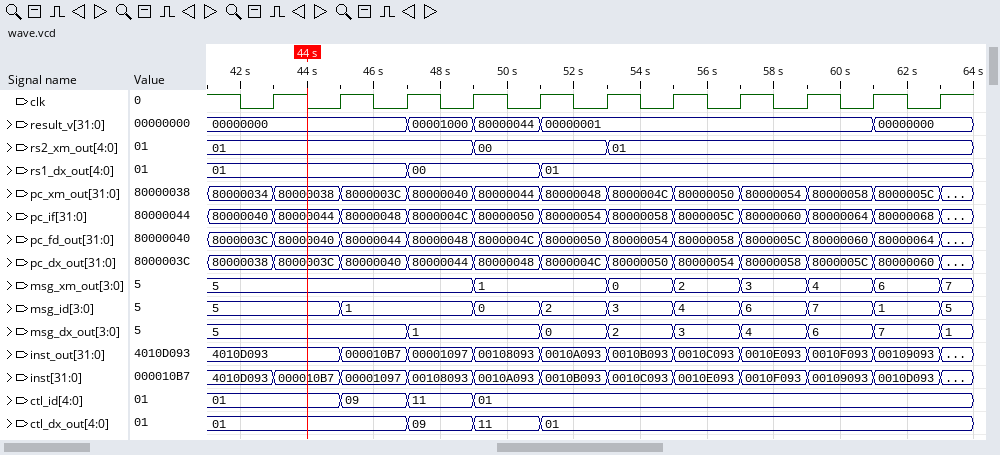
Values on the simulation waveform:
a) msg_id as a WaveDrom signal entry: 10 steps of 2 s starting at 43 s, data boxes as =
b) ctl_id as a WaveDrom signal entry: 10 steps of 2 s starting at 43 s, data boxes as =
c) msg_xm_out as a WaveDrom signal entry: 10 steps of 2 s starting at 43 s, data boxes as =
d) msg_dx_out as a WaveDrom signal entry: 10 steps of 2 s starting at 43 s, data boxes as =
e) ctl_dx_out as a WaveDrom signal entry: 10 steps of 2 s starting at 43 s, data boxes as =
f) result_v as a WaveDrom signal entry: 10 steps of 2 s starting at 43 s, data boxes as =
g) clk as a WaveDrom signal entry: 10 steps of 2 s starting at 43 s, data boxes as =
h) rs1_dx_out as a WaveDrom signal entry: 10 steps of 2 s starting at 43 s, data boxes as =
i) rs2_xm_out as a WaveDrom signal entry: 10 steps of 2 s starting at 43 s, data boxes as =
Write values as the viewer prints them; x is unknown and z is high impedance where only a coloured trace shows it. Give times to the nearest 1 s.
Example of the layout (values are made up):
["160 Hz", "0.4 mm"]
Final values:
["{name: 'msg_id', wave: '==.=======', data: '5 1 0 2 3 4 6 7 1'}", "{name: 'ctl_id', wave: '====......', data: '01 09 11 01'}", "{name: 'msg_xm_out', wave: '=..=.=====', data: '5 1 0 2 3 4 6'}", "{name: 'msg_dx_out', wave: '=.=.======', data: '5 1 0 2 3 4 6 7'}", "{name: 'ctl_dx_out', wave: '=.===.....', data: '01 09 11 01'}", "{name: 'result_v', wave: '=.===....=', data: '00000000 00001000 80000044 00000001 00000000'}", "{name: 'clk', wave: 'p.........'}", "{name: 'rs1_dx_out', wave: '=.=.=.....', data: '01 00 01'}", "{name: 'rs2_xm_out', wave: '=..=.=....', data: '01 00 01'}"]
